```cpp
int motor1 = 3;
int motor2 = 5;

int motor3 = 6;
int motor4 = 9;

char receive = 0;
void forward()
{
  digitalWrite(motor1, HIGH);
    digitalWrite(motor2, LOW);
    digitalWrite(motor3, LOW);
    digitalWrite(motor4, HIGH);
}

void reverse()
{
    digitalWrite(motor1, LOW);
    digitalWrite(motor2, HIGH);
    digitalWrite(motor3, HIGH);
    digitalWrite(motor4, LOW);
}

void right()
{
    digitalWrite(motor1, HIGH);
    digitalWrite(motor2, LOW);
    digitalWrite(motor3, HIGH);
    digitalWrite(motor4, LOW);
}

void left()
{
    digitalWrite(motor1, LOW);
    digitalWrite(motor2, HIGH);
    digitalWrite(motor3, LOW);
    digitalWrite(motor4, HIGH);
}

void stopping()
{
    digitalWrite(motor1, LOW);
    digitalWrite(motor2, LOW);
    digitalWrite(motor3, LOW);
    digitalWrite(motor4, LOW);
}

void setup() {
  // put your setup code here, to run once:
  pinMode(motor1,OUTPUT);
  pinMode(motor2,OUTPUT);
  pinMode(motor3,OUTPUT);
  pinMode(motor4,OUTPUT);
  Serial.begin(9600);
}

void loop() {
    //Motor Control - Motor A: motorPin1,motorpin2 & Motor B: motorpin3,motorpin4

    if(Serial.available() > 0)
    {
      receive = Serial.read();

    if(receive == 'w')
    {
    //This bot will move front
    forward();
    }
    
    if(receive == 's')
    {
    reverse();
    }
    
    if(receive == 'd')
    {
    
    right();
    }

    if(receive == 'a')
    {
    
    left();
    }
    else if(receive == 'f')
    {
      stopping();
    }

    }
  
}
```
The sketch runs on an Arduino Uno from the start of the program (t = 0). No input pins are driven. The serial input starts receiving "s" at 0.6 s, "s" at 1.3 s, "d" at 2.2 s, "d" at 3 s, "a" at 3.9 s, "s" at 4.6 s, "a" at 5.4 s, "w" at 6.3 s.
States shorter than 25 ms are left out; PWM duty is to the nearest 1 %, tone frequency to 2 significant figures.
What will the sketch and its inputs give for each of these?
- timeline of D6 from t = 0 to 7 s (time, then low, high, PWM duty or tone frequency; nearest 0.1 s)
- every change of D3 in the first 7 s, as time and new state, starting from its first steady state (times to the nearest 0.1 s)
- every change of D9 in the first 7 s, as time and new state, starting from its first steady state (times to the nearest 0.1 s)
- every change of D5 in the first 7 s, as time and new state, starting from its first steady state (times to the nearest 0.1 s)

0 s low; 0.6 s high; 3.9 s low; 4.6 s high; 5.4 s low
0 s low; 2.2 s high; 3.9 s low; 6.3 s high
0 s low; 3.9 s high; 4.6 s low; 5.4 s high
0 s low; 0.6 s high; 2.2 s low; 3.9 s high; 6.3 s low
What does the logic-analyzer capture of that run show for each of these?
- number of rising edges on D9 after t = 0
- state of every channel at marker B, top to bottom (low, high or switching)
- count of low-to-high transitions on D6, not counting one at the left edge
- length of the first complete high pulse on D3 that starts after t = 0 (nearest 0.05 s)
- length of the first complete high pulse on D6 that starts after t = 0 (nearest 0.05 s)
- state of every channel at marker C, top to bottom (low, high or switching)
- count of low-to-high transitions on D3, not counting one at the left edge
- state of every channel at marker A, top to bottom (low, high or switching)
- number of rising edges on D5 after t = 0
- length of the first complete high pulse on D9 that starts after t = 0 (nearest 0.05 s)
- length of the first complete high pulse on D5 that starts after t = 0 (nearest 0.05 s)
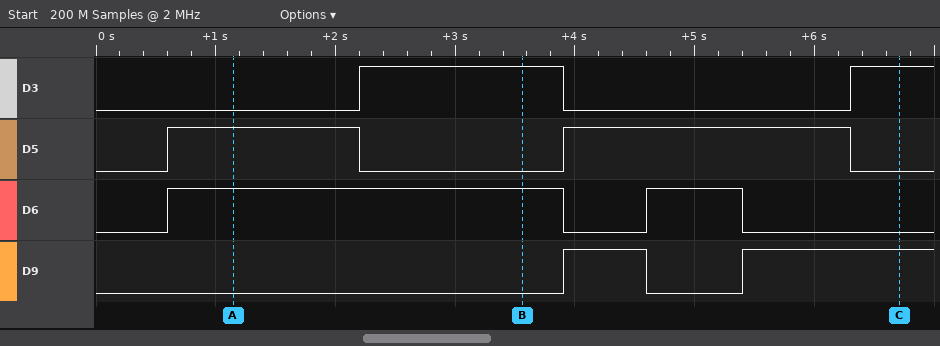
2
D3 high, D5 low, D6 high, D9 low
2
1.70 s
3.30 s
D3 high, D5 low, D6 low, D9 high
2
D3 low, D5 high, D6 high, D9 low
2
0.70 s
1.60 s
